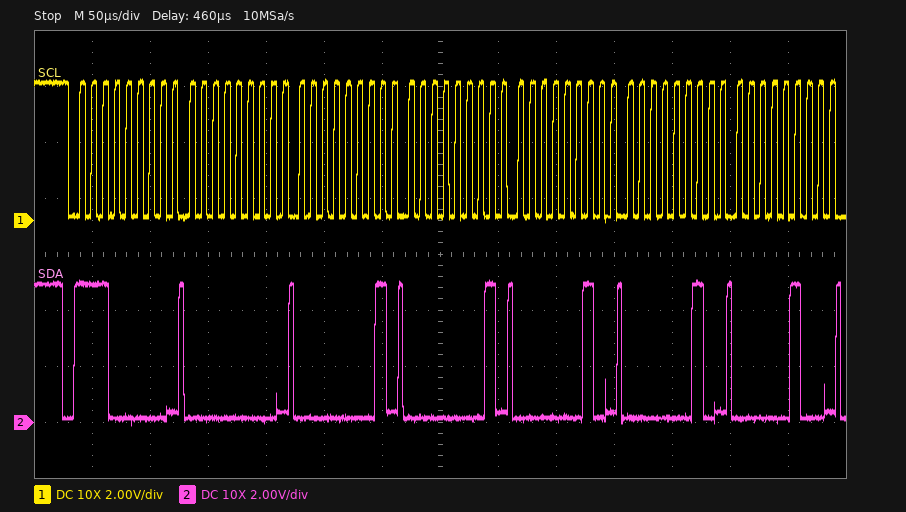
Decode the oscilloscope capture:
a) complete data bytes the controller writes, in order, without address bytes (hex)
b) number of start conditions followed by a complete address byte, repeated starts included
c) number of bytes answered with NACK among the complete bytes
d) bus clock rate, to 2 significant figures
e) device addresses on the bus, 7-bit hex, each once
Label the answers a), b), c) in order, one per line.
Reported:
a) 00 01 01 02 02 04
b) 1
c) 0
d) 100 kHz
e) 0x70
